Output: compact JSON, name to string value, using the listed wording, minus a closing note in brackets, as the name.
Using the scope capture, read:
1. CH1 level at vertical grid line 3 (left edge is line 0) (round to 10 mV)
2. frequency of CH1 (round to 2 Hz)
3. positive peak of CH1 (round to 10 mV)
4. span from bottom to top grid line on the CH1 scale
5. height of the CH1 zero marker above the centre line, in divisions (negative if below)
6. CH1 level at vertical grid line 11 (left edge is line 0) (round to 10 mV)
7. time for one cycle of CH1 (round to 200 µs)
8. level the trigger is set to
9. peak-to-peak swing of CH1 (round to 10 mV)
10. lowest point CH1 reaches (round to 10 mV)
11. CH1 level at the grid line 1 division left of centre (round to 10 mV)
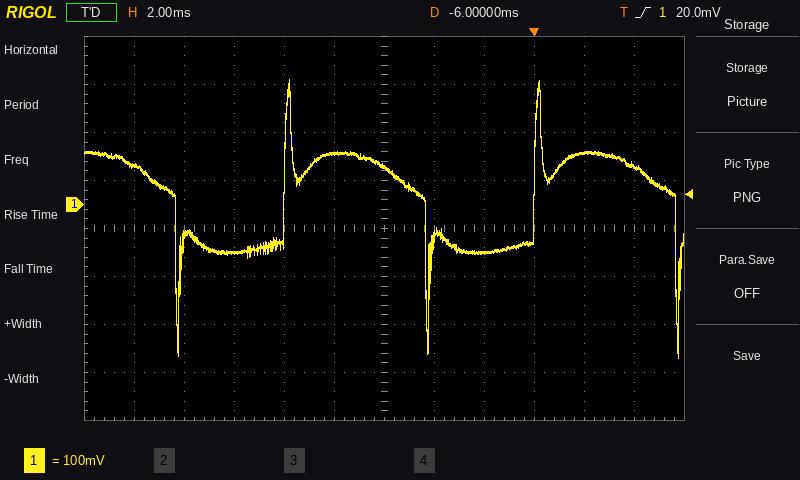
{"CH1 level at vertical grid line 3 (left edge is line 0)": "-100 mV", "frequency of CH1": "100 Hz", "positive peak of CH1": "260 mV", "span from bottom to top grid line on the CH1 scale": "800 mV", "height of the CH1 zero marker above the centre line, in divisions": "+0.5 div", "CH1 level at vertical grid line 11 (left edge is line 0)": "80 mV", "time for one cycle of CH1": "10.0 ms", "level the trigger is set to": "20.0 mV", "peak-to-peak swing of CH1": "580 mV", "lowest point CH1 reaches": "-320 mV", "CH1 level at the grid line 1 division left of centre": "110 mV"}
